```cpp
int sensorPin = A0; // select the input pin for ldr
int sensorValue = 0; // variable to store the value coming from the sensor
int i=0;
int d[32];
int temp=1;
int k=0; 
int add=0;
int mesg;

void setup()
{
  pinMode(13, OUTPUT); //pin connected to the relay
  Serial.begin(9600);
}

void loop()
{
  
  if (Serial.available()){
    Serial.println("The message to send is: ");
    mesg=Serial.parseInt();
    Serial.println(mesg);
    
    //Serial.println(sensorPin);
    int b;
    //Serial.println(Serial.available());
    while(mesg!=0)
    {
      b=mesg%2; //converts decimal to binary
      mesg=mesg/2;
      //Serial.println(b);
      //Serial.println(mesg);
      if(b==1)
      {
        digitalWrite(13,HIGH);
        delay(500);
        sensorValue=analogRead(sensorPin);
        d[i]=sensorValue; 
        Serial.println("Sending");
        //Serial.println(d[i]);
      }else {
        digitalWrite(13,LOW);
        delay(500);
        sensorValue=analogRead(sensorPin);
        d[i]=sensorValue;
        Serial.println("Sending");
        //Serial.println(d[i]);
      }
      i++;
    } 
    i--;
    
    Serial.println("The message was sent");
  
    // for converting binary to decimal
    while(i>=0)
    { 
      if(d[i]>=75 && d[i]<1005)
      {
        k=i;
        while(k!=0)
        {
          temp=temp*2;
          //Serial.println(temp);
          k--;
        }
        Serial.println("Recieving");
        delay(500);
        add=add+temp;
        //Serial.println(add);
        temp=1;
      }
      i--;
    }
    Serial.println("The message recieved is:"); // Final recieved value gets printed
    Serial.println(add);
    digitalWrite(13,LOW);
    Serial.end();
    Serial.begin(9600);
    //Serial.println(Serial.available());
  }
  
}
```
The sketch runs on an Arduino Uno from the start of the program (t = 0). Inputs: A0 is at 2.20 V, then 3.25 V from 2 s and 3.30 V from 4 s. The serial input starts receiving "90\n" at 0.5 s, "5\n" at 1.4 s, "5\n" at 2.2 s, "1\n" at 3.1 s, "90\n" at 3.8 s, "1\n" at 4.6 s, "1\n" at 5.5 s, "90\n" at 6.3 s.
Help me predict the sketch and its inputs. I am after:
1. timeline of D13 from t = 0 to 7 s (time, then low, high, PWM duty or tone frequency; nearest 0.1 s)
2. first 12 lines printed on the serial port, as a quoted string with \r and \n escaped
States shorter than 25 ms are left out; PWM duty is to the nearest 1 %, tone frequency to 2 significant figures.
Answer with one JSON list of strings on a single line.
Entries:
["0 s low; 1 s high; 1.5 s low; 2 s high; 3 s low; 3.5 s high", "\"The message to send is: \\r\\n90\\r\\nSending\\r\\nSending\\r\\nSending\\r\\nSending\\r\\nSending\\r\\nSending\\r\\nSending\\r\\nThe message was sent\\r\\nRecieving\\r\\nRecieving\\r\\n\""]
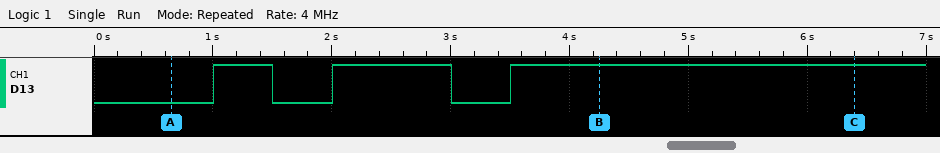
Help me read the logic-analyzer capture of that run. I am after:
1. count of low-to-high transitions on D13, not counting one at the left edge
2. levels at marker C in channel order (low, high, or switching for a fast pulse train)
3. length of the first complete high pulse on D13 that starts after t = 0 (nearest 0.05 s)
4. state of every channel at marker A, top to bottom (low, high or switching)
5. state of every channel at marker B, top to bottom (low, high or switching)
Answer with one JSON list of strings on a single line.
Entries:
["3", "D13 high", "0.50 s", "D13 low", "D13 high"]
